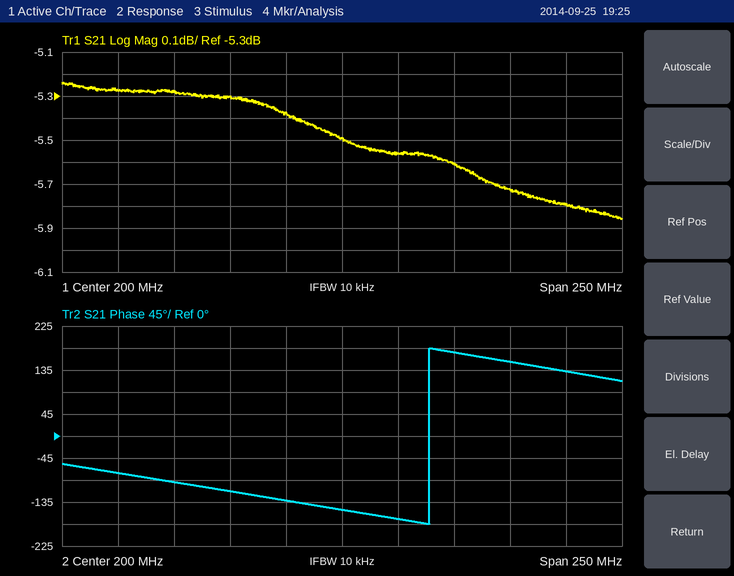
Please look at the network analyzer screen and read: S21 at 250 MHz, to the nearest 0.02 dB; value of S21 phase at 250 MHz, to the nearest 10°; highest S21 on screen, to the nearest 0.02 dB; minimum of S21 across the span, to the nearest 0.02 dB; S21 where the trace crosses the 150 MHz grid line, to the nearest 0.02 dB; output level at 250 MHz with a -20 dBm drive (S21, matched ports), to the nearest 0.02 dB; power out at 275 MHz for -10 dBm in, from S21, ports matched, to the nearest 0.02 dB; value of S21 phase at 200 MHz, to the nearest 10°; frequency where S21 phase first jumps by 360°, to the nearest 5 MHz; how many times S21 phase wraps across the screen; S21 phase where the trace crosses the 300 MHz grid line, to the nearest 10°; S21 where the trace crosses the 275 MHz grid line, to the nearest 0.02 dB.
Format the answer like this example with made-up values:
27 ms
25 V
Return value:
-5.60 dB
170°
-5.24 dB
-5.86 dB
-5.30 dB
-25.60 dBm
-15.72 dBm
-150°
240 MHz
1
130°
-5.72 dB
